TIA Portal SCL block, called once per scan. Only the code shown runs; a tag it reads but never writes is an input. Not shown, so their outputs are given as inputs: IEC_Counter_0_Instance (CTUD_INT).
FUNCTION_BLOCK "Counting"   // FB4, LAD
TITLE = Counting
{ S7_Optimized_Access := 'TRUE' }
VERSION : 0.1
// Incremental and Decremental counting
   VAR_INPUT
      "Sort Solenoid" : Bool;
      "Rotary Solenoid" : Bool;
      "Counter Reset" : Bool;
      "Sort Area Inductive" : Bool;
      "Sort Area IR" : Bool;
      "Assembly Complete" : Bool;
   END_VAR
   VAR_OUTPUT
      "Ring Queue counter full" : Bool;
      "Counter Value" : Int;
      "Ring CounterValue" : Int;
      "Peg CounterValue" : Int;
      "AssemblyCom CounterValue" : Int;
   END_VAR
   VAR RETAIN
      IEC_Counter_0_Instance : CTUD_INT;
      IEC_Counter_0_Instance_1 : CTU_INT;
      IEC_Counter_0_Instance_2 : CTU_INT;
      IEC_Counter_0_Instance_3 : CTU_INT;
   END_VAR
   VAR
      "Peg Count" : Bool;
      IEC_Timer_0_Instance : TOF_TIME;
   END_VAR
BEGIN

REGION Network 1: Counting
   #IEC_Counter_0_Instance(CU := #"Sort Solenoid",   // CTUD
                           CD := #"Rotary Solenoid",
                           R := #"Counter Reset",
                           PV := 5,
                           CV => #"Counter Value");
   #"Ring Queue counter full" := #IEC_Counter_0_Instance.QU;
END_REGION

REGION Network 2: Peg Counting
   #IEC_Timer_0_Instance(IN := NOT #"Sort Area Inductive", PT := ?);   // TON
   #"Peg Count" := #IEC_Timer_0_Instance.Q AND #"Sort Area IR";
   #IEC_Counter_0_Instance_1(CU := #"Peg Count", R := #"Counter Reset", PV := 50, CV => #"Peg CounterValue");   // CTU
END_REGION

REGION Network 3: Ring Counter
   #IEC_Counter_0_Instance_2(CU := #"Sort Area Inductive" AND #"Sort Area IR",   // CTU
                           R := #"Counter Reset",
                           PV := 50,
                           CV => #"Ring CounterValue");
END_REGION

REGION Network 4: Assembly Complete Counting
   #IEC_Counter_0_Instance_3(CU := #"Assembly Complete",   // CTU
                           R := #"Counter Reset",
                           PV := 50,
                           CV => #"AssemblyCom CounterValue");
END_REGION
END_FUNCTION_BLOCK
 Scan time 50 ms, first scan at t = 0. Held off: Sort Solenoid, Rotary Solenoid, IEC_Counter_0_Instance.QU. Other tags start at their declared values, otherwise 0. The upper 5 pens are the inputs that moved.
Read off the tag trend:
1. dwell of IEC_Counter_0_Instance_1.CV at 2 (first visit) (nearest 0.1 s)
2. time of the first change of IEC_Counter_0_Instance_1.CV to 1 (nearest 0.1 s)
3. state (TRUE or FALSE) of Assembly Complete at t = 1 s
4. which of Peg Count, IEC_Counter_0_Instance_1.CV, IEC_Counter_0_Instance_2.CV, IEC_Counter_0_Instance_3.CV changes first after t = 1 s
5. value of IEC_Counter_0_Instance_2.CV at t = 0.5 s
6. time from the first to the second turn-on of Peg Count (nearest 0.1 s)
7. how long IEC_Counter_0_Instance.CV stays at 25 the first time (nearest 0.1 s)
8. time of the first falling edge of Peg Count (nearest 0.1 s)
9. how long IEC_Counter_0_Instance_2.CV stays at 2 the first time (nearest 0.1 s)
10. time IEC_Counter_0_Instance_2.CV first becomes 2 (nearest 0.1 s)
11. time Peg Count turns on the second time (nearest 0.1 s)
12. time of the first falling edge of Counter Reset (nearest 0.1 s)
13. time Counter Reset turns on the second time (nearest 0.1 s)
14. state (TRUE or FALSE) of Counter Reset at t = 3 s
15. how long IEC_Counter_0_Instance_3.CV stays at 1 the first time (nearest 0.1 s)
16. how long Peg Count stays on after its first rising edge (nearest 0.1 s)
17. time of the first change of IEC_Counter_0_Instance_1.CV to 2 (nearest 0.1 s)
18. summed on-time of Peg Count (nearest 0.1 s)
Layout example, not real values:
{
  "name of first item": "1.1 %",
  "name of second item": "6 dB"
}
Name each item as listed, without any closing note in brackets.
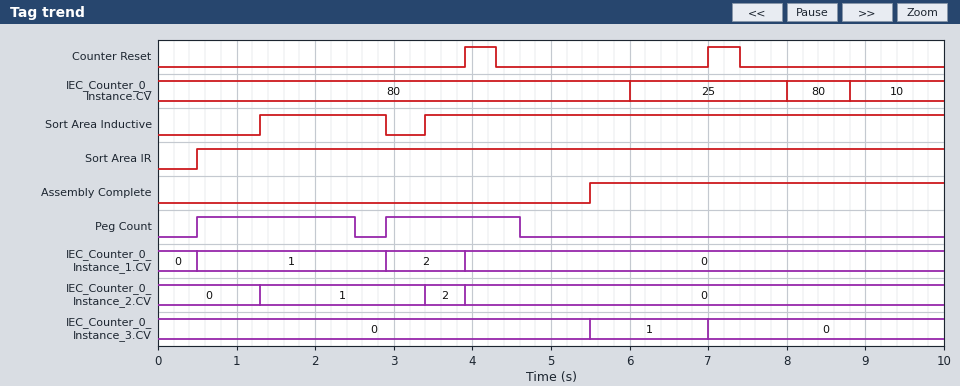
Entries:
{
  "dwell of IEC_Counter_0_Instance_1.CV at 2 (first visit)": "1.0 s",
  "time of the first change of IEC_Counter_0_Instance_1.CV to 1": "0.5 s",
  "state (TRUE or FALSE) of Assembly Complete at t = 1 s": "FALSE",
  "which of Peg Count, IEC_Counter_0_Instance_1.CV, IEC_Counter_0_Instance_2.CV, IEC_Counter_0_Instance_3.CV changes first after t = 1 s": "IEC_Counter_0_Instance_2.CV",
  "value of IEC_Counter_0_Instance_2.CV at t = 0.5 s": "0",
  "time from the first to the second turn-on of Peg Count": "2.4 s",
  "how long IEC_Counter_0_Instance.CV stays at 25 the first time": "2.0 s",
  "time of the first falling edge of Peg Count": "2.5 s",
  "how long IEC_Counter_0_Instance_2.CV stays at 2 the first time": "0.5 s",
  "time IEC_Counter_0_Instance_2.CV first becomes 2": "3.4 s",
  "time Peg Count turns on the second time": "2.9 s",
  "time of the first falling edge of Counter Reset": "4.3 s",
  "time Counter Reset turns on the second time": "7.0 s",
  "state (TRUE or FALSE) of Counter Reset at t = 3 s": "FALSE",
  "how long IEC_Counter_0_Instance_3.CV stays at 1 the first time": "1.5 s",
  "how long Peg Count stays on after its first rising edge": "2.0 s",
  "time of the first change of IEC_Counter_0_Instance_1.CV to 2": "2.9 s",
  "summed on-time of Peg Count": "3.7 s"
}
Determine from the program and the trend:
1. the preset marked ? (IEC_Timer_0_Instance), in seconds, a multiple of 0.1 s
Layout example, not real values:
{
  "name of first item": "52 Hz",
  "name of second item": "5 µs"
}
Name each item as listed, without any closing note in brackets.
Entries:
{
  "the preset marked ? (IEC_Timer_0_Instance), in seconds, a multiple of 0.1 s": "1.2 s"
}
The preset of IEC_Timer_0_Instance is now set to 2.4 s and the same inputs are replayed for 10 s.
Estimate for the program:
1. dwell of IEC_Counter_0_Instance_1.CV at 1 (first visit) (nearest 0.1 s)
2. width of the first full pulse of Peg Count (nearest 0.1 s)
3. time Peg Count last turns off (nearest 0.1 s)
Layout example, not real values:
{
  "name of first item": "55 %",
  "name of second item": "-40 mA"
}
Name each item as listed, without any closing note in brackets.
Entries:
{
  "dwell of IEC_Counter_0_Instance_1.CV at 1 (first visit)": "3.4 s",
  "width of the first full pulse of Peg Count": "5.3 s",
  "time Peg Count last turns off": "5.8 s"
}
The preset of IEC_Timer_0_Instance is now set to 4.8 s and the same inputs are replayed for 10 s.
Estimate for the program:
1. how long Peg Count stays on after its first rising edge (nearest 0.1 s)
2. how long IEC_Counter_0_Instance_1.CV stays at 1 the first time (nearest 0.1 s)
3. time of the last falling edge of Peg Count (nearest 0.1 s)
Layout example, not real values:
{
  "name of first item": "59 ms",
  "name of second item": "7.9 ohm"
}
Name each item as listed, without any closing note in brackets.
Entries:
{
  "how long Peg Count stays on after its first rising edge": "7.7 s",
  "how long IEC_Counter_0_Instance_1.CV stays at 1 the first time": "3.4 s",
  "time of the last falling edge of Peg Count": "8.2 s"
}
